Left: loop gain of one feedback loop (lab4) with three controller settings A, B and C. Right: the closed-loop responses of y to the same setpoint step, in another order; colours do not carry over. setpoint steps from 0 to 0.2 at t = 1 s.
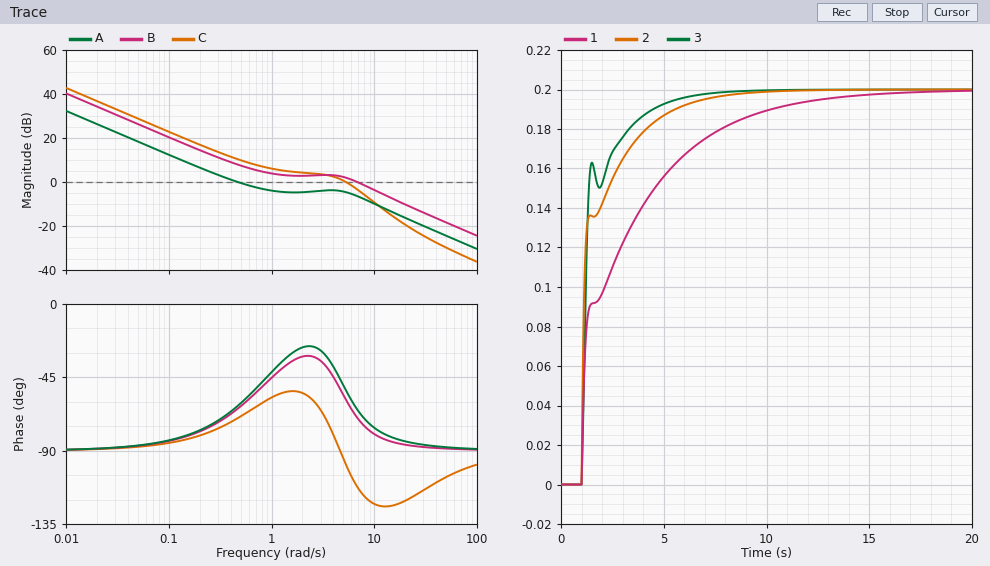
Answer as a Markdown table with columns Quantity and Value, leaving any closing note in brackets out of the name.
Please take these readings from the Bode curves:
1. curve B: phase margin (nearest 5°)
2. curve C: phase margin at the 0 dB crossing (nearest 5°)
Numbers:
| Quantity | Value |
|---|---|
| curve B: phase margin | 110° |
| curve C: phase margin at the 0 dB crossing | 80° |
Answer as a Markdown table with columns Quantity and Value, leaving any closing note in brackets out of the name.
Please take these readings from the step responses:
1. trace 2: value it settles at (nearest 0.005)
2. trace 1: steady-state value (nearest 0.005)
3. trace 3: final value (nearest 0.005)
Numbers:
| Quantity | Value |
|---|---|
| trace 2: value it settles at | 0.200 |
| trace 1: steady-state value | 0.200 |
| trace 3: final value | 0.200 |
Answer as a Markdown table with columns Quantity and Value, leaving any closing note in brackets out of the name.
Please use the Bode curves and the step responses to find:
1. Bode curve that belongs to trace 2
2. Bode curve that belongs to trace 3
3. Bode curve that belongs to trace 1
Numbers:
| Quantity | Value |
|---|---|
| Bode curve that belongs to trace 2 | B |
| Bode curve that belongs to trace 3 | C |
| Bode curve that belongs to trace 1 | A |
